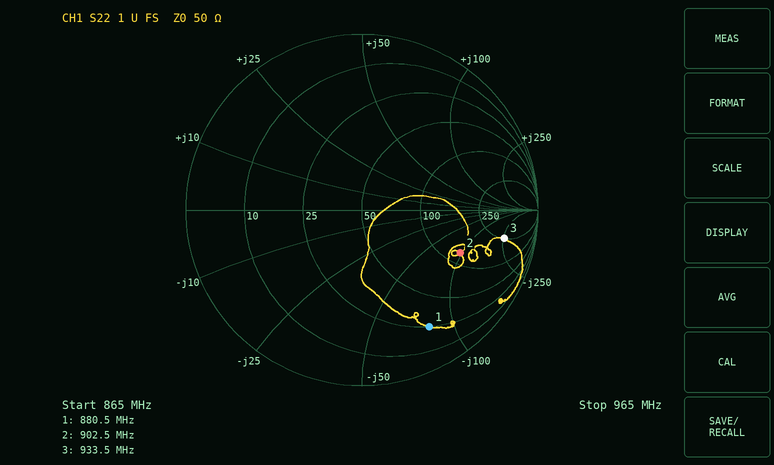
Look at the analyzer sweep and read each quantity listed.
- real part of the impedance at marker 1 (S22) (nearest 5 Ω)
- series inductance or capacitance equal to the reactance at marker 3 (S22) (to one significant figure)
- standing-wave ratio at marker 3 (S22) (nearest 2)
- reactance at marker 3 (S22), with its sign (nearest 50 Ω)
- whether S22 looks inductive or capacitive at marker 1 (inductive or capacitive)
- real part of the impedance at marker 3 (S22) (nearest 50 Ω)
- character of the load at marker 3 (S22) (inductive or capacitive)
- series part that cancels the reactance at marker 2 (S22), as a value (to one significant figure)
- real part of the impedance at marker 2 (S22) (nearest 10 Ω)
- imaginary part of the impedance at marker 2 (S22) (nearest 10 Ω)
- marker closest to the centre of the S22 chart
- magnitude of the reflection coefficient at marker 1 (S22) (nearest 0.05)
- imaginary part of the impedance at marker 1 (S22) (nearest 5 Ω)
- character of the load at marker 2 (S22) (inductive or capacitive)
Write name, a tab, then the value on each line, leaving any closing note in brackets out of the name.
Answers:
real part of the impedance at marker 1 (S22)	25 Ω
series inductance or capacitance equal to the reactance at marker 3 (S22)	700 fF
standing-wave ratio at marker 3 (S22)	10
reactance at marker 3 (S22), with its sign	-250 Ω
whether S22 looks inductive or capacitive at marker 1	capacitive
real part of the impedance at marker 3 (S22)	250 Ω
character of the load at marker 3 (S22)	capacitive
series part that cancels the reactance at marker 2 (S22), as a value	20 nH
real part of the impedance at marker 2 (S22)	120 Ω
imaginary part of the impedance at marker 2 (S22)	-100 Ω
marker closest to the centre of the S22 chart	marker 2
magnitude of the reflection coefficient at marker 1 (S22)	0.75
imaginary part of the impedance at marker 1 (S22)	-80 Ω
character of the load at marker 2 (S22)	capacitive
